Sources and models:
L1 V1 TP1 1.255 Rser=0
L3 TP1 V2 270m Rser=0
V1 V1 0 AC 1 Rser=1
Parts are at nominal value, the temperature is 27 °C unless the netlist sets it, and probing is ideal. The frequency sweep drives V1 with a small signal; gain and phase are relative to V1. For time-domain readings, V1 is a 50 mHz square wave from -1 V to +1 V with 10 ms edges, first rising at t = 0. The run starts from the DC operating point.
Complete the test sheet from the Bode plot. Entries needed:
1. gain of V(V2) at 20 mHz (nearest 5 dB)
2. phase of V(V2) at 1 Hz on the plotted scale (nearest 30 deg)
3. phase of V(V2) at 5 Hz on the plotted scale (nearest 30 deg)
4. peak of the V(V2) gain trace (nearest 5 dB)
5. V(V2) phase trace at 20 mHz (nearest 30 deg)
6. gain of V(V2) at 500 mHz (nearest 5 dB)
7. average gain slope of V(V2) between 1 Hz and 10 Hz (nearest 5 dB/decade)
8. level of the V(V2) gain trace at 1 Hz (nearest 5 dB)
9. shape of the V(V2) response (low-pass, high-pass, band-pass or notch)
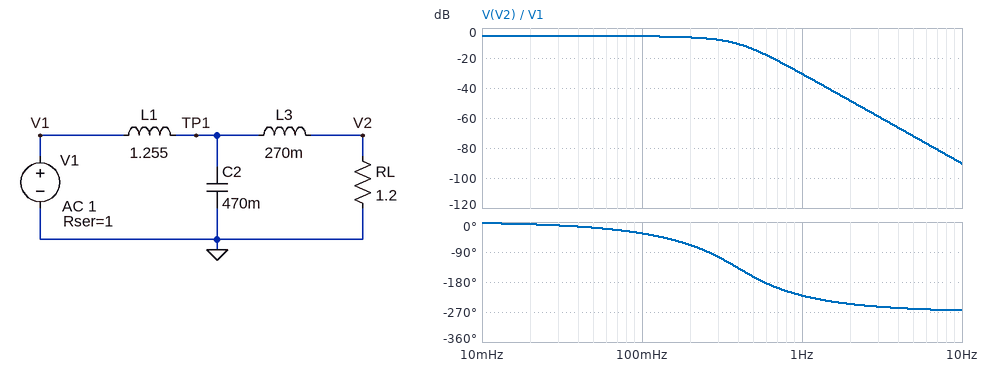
-5 dB
-210 deg
-270 deg
-5 dB
0 deg
-15 dB
-60 dB/decade
-30 dB
low-pass
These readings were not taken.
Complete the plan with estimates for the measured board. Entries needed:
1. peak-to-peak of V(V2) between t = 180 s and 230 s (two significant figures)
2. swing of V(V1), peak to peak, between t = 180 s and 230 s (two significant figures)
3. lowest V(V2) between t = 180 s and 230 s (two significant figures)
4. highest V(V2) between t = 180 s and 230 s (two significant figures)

1.1 V
2.9 V
-570 mV
570 mV
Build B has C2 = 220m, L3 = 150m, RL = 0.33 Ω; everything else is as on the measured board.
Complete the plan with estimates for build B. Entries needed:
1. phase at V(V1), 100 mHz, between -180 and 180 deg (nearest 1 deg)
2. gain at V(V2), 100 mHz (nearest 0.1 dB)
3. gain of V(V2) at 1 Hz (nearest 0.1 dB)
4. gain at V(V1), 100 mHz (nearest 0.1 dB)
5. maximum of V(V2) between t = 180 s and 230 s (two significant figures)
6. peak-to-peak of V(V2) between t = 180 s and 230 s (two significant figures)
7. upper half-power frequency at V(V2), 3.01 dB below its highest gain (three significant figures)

36 deg
-13.6 dB
-21.0 dB
-4.7 dB
250 mV
500 mV
160 mHz
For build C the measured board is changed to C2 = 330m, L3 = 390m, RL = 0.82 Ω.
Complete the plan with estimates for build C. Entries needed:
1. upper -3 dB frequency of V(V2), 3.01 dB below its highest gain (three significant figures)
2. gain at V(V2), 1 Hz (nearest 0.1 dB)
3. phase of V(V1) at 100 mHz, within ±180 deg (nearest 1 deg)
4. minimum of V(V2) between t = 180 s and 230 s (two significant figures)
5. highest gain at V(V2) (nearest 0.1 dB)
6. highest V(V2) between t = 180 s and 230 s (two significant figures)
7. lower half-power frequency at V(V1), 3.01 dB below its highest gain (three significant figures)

439 mHz
-32.0 dB
20 deg
-450 mV
-6.9 dB
450 mV
161 mHz
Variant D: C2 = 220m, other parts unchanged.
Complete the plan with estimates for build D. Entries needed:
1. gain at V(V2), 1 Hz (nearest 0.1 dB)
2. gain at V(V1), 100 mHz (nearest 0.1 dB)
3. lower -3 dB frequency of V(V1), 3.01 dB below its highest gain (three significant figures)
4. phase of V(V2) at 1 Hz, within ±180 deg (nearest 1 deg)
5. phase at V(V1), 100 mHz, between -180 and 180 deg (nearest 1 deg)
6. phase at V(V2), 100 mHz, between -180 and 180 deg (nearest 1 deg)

-22.0 dB
-4.3 dB
187 mHz
151 deg
13 deg
-28 deg
